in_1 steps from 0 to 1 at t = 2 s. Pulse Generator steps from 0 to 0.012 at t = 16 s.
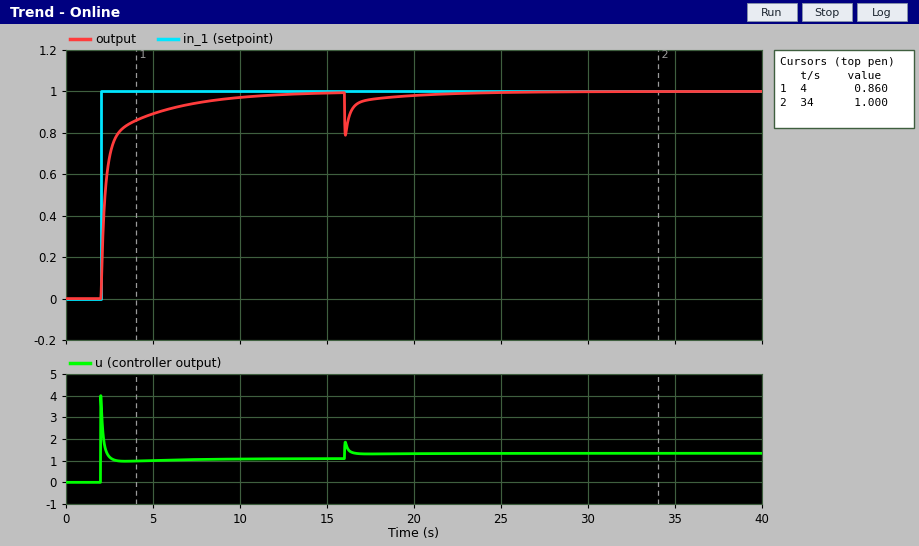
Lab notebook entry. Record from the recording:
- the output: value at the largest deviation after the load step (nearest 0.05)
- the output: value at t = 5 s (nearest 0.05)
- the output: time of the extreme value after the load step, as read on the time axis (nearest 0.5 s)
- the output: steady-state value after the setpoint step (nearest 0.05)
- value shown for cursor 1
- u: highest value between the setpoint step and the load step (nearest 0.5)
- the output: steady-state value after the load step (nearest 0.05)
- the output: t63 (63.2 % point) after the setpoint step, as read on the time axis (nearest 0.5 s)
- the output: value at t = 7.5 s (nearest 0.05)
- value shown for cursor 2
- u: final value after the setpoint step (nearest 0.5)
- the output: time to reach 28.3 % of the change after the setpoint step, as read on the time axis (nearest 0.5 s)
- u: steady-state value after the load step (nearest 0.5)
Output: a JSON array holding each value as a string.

["0.80", "0.90", "16.0 s", "1.00", "0.860", "4.0", "1.00", "2.5 s", "0.95", "1.000", "1.0", "2.0 s", "1.5"]
